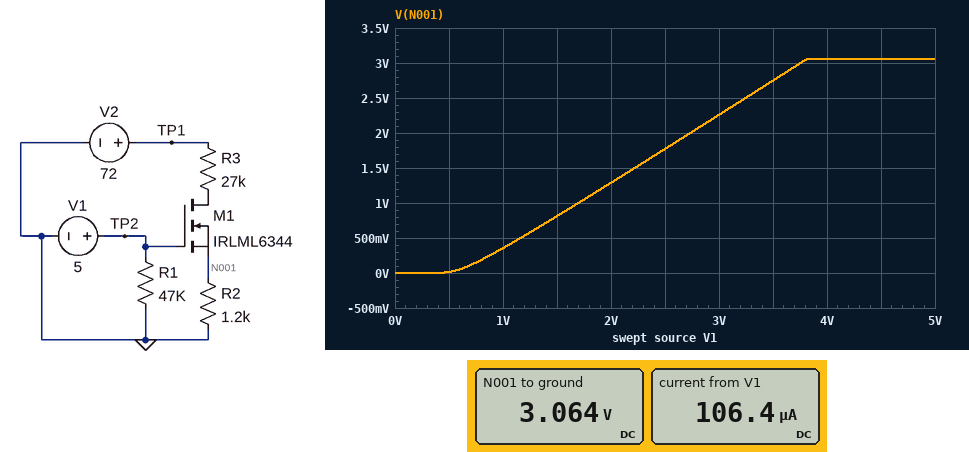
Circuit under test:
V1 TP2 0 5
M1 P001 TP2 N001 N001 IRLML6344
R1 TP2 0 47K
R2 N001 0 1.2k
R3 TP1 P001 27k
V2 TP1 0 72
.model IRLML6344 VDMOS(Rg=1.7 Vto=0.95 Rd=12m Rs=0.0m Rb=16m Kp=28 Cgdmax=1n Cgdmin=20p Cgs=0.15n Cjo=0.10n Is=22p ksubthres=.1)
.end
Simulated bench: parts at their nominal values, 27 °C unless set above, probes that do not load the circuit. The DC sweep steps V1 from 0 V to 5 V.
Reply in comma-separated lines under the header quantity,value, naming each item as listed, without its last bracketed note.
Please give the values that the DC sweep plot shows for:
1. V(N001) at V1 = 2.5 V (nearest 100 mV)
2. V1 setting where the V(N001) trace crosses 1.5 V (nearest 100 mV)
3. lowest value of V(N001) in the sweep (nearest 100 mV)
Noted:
quantity,value
V(N001) at V1 = 2.5 V,1.8 V
V1 setting where the V(N001) trace crosses 1.5 V,2.2 V
lowest value of V(N001) in the sweep,0 V
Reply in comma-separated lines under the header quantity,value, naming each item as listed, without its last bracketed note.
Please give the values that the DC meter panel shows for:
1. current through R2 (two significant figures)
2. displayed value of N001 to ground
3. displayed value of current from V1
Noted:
quantity,value
current through R2,2.6 mA
displayed value of N001 to ground,3.064 V
displayed value of current from V1,106.4 µA
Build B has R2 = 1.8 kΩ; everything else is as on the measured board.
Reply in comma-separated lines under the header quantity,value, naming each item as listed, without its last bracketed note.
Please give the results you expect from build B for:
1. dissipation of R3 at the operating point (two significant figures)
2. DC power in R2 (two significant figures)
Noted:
quantity,value
dissipation of R3 at the operating point,150 mW
DC power in R2,10 mW
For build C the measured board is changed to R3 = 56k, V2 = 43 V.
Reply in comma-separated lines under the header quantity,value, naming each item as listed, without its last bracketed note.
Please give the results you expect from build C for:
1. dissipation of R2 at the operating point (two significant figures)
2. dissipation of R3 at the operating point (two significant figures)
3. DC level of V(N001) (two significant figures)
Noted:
quantity,value
dissipation of R2 at the operating point,680 µW
dissipation of R3 at the operating point,32 mW
DC level of V(N001),900 mV
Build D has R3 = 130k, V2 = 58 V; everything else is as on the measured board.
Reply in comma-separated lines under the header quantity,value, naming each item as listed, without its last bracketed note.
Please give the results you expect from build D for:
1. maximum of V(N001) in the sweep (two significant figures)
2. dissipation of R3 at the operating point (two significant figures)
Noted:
quantity,value
maximum of V(N001) in the sweep,530 mV
dissipation of R3 at the operating point,25 mW
